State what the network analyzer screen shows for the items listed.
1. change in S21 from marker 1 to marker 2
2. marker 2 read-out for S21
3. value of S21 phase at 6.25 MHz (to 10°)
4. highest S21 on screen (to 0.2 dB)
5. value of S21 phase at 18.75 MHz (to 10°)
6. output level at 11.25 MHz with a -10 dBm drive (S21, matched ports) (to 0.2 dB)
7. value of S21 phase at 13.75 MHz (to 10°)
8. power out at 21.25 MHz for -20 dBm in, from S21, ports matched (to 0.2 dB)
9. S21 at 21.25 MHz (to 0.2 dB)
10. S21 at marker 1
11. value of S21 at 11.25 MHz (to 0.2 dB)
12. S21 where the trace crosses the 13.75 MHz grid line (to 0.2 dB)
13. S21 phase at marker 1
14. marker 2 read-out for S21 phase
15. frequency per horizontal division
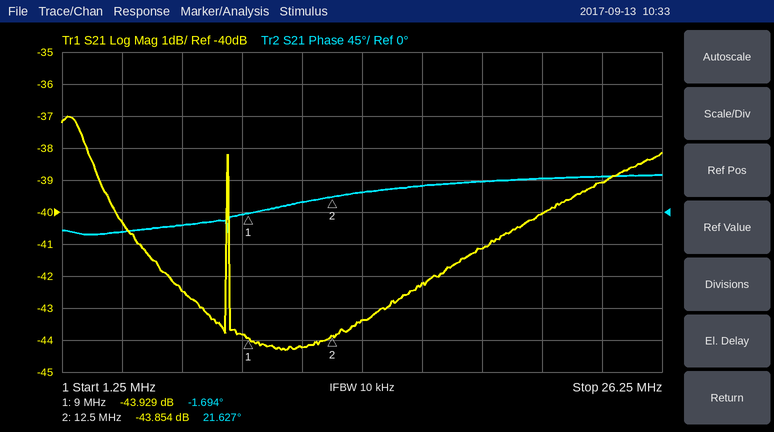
0.075 dB
-43.854 dB
-20°
-37.0 dB
40°
-54.2 dBm
30°
-60.0 dBm
-40.0 dB
-43.929 dB
-44.2 dB
-43.4 dB
-1.694°
21.627°
2.5 MHz
